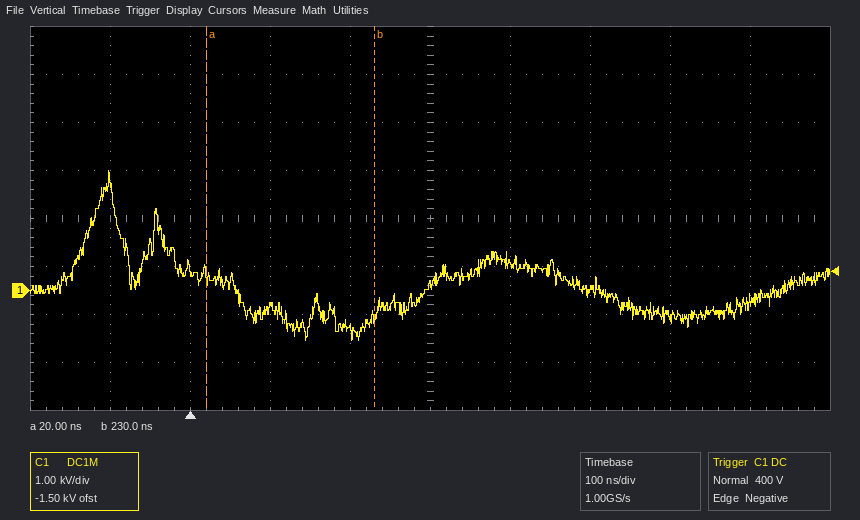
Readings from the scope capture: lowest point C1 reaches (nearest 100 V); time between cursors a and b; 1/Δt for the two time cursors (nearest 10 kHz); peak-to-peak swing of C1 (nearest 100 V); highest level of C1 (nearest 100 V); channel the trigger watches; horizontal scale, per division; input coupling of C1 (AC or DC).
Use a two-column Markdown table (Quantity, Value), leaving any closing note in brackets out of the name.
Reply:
| Quantity | Value |
|---|---|
| lowest point C1 reaches | -1.0 kV |
| time between cursors a and b | 210 ns |
| 1/Δt for the two time cursors | 4.76 MHz |
| peak-to-peak swing of C1 | 3.5 kV |
| highest level of C1 | 2.5 kV |
| channel the trigger watches | C1 |
| horizontal scale, per division | 100 ns |
| input coupling of C1 | DC |
